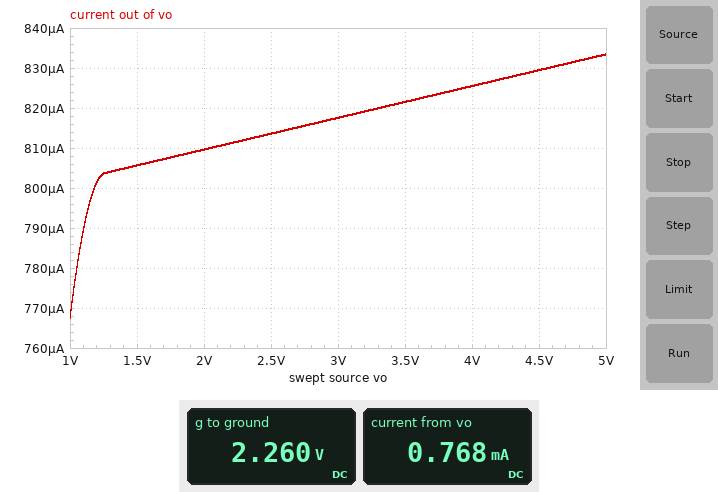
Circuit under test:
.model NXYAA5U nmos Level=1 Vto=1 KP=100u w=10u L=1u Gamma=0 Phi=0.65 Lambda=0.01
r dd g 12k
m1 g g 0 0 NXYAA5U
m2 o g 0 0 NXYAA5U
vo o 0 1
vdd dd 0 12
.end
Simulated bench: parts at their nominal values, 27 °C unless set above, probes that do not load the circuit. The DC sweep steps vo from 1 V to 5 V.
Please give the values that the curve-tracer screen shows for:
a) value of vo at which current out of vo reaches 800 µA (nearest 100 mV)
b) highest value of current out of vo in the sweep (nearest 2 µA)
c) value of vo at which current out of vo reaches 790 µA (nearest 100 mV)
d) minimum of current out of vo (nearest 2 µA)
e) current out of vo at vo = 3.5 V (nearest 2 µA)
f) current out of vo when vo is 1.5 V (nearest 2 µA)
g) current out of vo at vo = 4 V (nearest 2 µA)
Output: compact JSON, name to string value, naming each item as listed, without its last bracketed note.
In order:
{"value of vo at which current out of vo reaches 800 µA": "1.2 V", "highest value of current out of vo in the sweep": "834 µA", "value of vo at which current out of vo reaches 790 µA": "1.1 V", "minimum of current out of vo": "768 µA", "current out of vo at vo = 3.5 V": "822 µA", "current out of vo when vo is 1.5 V": "806 µA", "current out of vo at vo = 4 V": "826 µA"}
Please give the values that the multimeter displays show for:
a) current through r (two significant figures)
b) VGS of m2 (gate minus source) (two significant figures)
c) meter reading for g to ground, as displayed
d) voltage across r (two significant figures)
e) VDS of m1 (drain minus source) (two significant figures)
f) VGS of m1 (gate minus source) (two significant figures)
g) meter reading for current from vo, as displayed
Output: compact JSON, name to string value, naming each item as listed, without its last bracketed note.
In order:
{"current through r": "810 µA", "VGS of m2 (gate minus source)": "2.3 V", "meter reading for g to ground, as displayed": "2.260 V", "voltage across r": "9.7 V", "VDS of m1 (drain minus source)": "2.3 V", "VGS of m1 (gate minus source)": "2.3 V", "meter reading for current from vo, as displayed": "0.768 mA"}
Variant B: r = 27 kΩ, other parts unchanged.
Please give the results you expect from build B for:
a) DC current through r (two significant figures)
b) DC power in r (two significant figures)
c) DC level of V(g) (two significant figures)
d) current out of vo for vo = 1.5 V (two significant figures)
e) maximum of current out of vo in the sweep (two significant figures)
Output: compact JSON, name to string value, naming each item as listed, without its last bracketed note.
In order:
{"DC current through r": "380 µA", "DC power in r": "3.8 mW", "DC level of V(g)": "1.9 V", "current out of vo for vo = 1.5 V": "370 µA", "maximum of current out of vo in the sweep": "390 µA"}
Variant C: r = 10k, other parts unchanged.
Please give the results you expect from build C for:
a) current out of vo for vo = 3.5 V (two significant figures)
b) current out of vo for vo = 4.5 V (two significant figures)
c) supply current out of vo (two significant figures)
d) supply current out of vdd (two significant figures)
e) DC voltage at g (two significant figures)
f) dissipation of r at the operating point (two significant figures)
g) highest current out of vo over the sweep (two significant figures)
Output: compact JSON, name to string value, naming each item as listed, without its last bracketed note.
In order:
{"current out of vo for vo = 3.5 V": "970 µA", "current out of vo for vo = 4.5 V": "980 µA", "supply current out of vo": "880 µA", "supply current out of vdd": "960 µA", "DC voltage at g": "2.4 V", "dissipation of r at the operating point": "9.3 mW", "highest current out of vo over the sweep": "990 µA"}
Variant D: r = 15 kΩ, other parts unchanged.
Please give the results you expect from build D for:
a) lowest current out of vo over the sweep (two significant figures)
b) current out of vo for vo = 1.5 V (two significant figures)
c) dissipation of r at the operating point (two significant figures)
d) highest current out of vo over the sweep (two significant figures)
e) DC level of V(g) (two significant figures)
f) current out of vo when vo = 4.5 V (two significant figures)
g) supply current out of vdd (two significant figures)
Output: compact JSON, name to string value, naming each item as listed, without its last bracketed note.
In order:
{"lowest current out of vo over the sweep": "640 µA", "current out of vo for vo = 1.5 V": "650 µA", "dissipation of r at the operating point": "6.5 mW", "highest current out of vo over the sweep": "680 µA", "DC level of V(g)": "2.1 V", "current out of vo when vo = 4.5 V": "670 µA", "supply current out of vdd": "660 µA"}
